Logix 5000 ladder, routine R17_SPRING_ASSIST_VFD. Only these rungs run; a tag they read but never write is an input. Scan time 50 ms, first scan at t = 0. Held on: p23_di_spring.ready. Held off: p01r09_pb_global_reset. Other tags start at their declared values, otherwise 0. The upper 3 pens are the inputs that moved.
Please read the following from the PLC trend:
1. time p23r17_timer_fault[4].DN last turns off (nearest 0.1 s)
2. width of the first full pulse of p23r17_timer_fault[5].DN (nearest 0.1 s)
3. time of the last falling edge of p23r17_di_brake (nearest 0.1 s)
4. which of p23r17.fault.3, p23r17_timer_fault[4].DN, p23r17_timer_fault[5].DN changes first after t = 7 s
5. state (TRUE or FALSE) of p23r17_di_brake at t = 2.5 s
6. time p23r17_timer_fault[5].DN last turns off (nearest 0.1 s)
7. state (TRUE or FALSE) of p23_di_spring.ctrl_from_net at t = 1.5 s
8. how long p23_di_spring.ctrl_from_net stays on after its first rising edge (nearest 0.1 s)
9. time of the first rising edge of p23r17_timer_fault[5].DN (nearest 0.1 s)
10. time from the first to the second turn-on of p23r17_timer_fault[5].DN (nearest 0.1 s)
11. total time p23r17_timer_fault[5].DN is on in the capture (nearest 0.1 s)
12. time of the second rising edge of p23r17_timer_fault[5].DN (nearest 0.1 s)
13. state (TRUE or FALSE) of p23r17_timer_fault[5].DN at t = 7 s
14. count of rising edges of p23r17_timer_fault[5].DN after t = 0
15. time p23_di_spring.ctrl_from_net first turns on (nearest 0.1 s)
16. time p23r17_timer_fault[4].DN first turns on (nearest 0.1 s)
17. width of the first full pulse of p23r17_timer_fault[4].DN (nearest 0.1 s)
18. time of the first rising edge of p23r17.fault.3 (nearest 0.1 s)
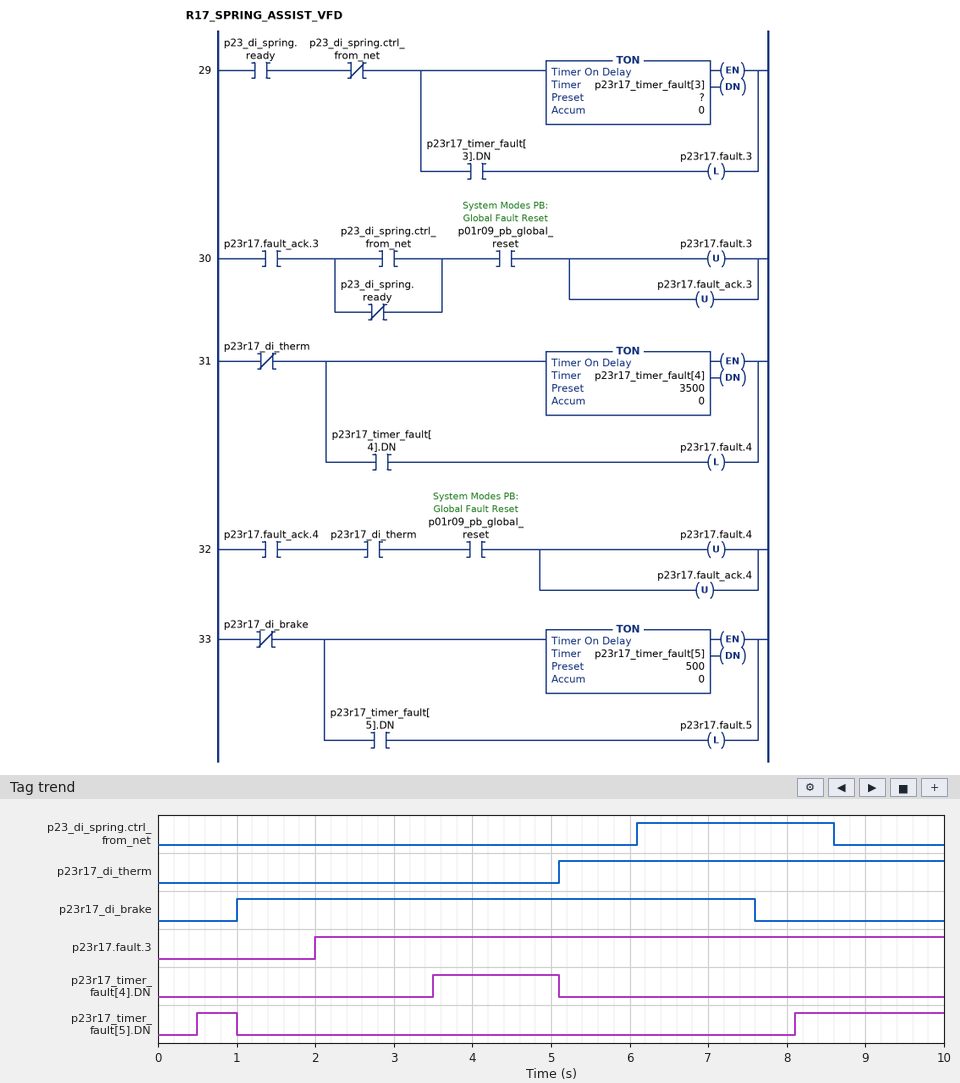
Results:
5.1 s
0.5 s
7.6 s
p23r17_timer_fault[5].DN
TRUE
1.0 s
FALSE
2.5 s
0.5 s
7.6 s
2.4 s
8.1 s
FALSE
2
6.1 s
3.5 s
1.6 s
2.0 s
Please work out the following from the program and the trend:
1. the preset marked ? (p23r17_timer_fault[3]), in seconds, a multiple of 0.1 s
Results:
2.0 s
